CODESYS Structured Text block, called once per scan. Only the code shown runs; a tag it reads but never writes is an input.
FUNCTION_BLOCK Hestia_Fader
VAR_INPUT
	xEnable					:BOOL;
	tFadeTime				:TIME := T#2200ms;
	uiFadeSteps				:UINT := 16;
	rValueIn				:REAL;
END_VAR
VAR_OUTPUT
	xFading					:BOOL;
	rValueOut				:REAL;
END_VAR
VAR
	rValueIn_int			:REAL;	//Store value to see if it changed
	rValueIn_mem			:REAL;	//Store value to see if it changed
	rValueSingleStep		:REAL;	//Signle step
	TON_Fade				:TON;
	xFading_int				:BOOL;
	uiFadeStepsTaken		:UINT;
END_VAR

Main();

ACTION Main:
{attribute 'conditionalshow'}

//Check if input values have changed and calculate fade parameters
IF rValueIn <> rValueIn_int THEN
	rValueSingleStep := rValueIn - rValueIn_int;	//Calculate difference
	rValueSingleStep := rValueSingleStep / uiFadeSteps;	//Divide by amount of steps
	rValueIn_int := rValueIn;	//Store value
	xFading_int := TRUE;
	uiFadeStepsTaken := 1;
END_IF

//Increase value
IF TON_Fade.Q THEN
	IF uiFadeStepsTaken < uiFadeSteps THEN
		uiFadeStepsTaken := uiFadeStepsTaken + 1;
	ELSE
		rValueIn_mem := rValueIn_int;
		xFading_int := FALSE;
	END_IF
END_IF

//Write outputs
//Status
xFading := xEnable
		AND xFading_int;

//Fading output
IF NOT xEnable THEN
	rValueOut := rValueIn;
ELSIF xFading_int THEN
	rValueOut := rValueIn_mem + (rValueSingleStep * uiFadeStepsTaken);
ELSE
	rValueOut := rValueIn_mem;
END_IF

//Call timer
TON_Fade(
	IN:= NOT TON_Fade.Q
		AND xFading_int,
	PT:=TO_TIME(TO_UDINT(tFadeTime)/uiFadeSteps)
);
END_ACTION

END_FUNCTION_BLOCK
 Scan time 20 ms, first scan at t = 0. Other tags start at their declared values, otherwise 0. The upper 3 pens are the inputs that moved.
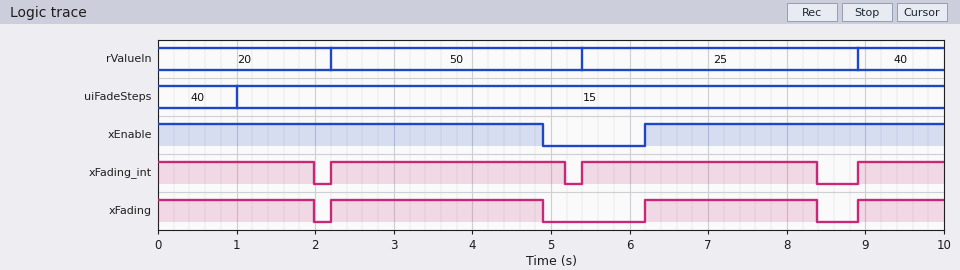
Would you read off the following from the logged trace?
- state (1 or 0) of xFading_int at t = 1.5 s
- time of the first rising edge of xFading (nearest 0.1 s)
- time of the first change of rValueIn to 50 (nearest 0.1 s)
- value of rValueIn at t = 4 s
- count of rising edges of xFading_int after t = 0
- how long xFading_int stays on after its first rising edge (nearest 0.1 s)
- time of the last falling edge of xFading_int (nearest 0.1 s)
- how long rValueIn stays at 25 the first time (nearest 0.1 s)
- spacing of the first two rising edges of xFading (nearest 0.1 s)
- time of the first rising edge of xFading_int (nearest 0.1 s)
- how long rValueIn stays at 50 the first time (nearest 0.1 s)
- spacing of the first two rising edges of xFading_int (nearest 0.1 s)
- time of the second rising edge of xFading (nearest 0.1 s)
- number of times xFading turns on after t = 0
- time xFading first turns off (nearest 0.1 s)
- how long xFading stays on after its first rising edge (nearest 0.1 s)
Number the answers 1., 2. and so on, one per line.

1. 1
2. 2.2 s
3. 2.2 s
4. 50
5. 3
6. 3.0 s
7. 8.4 s
8. 3.5 s
9. 4.0 s
10. 2.2 s
11. 3.2 s
12. 3.2 s
13. 6.2 s
14. 3
15. 2.0 s
16. 2.7 s
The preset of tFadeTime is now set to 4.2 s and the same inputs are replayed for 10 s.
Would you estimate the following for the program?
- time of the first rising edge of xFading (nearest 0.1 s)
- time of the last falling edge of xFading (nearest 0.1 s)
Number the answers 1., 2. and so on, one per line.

1. 6.2 s
2. 4.9 s
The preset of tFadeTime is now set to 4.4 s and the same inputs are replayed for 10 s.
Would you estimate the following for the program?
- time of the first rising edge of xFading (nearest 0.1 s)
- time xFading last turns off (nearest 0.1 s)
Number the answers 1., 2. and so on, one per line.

1. 6.2 s
2. 4.9 s
